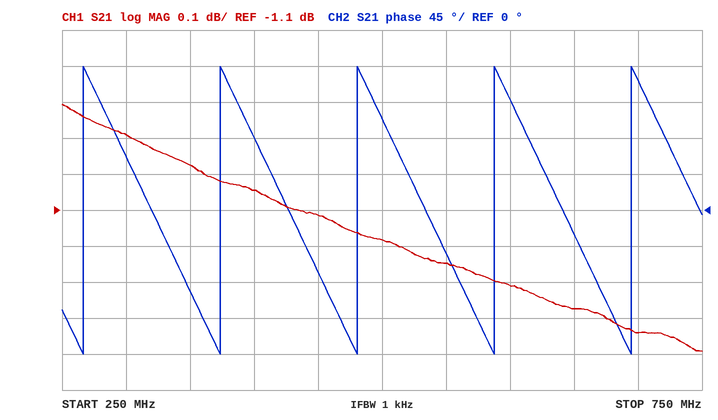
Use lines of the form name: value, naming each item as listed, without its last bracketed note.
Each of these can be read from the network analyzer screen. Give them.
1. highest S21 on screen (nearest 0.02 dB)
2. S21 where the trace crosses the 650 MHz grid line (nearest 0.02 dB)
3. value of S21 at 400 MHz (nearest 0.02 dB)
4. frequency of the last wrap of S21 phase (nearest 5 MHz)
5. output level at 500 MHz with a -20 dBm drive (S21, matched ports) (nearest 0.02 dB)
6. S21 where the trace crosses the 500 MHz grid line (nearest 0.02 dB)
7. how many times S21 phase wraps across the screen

highest S21 on screen: -0.80 dB
S21 where the trace crosses the 650 MHz grid line: -1.38 dB
value of S21 at 400 MHz: -1.04 dB
frequency of the last wrap of S21 phase: 695 MHz
output level at 500 MHz with a -20 dBm drive (S21, matched ports): -21.18 dBm
S21 where the trace crosses the 500 MHz grid line: -1.18 dB
how many times S21 phase wraps across the screen: 5
